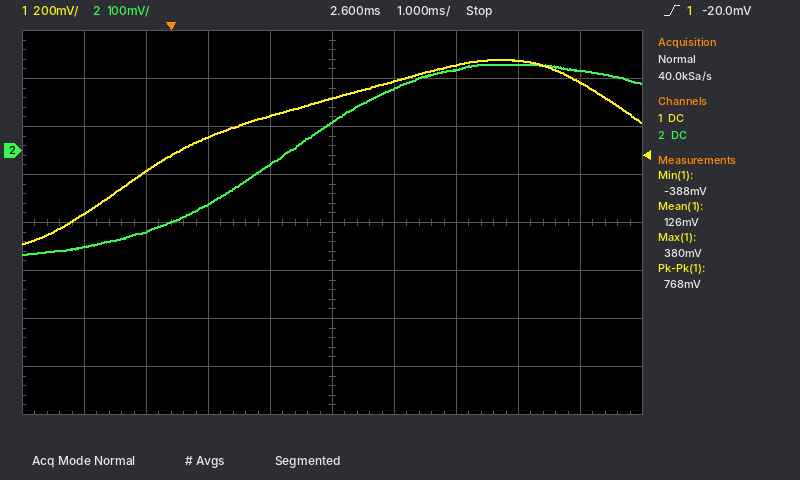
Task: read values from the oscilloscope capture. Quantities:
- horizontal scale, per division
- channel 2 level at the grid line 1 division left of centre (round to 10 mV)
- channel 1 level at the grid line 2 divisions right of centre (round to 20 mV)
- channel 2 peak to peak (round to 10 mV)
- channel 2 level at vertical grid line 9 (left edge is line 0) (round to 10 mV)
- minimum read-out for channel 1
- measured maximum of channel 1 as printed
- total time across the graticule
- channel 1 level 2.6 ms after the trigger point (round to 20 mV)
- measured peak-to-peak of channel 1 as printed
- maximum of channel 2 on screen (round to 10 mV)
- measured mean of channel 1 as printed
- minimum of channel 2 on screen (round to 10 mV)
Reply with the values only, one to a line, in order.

1 ms
-30 mV
360 mV
400 mV
170 mV
-388 mV
380 mV
10 ms
220 mV
768 mV
180 mV
126 mV
-220 mV
